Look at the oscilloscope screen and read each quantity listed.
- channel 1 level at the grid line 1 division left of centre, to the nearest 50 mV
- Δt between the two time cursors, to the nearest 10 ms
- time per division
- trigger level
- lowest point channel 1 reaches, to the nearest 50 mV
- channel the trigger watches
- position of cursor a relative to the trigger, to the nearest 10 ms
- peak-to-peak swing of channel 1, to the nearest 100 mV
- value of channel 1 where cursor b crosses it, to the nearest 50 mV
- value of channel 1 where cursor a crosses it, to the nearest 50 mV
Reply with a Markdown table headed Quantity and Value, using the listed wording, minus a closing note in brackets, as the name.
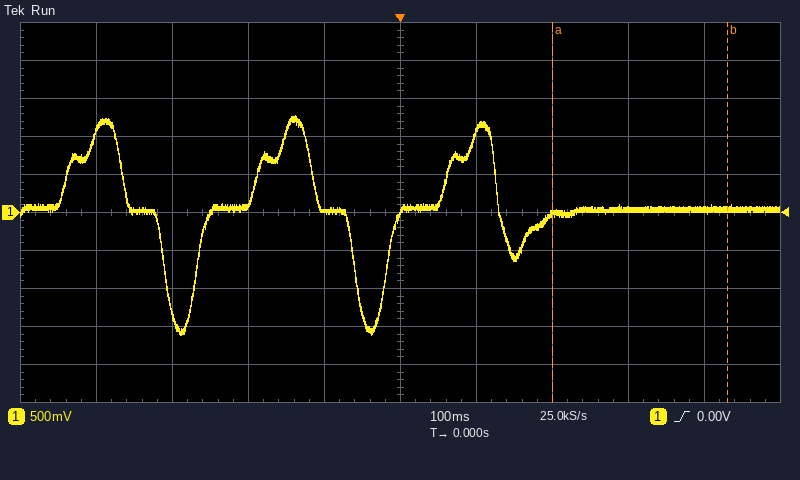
| Quantity | Value |
|---|---|
| channel 1 level at the grid line 1 division left of centre, to the nearest 50 mV | 50 mV |
| Δt between the two time cursors, to the nearest 10 ms | 230 ms |
| time per division | 100 ms |
| trigger level | 0.00 V |
| lowest point channel 1 reaches, to the nearest 50 mV | -1.60 V |
| channel the trigger watches | channel 1 |
| position of cursor a relative to the trigger, to the nearest 10 ms | +200 ms |
| peak-to-peak swing of channel 1, to the nearest 100 mV | 2.90 V |
| value of channel 1 where cursor b crosses it, to the nearest 50 mV | 50 mV |
| value of channel 1 where cursor a crosses it, to the nearest 50 mV | -50 mV |
